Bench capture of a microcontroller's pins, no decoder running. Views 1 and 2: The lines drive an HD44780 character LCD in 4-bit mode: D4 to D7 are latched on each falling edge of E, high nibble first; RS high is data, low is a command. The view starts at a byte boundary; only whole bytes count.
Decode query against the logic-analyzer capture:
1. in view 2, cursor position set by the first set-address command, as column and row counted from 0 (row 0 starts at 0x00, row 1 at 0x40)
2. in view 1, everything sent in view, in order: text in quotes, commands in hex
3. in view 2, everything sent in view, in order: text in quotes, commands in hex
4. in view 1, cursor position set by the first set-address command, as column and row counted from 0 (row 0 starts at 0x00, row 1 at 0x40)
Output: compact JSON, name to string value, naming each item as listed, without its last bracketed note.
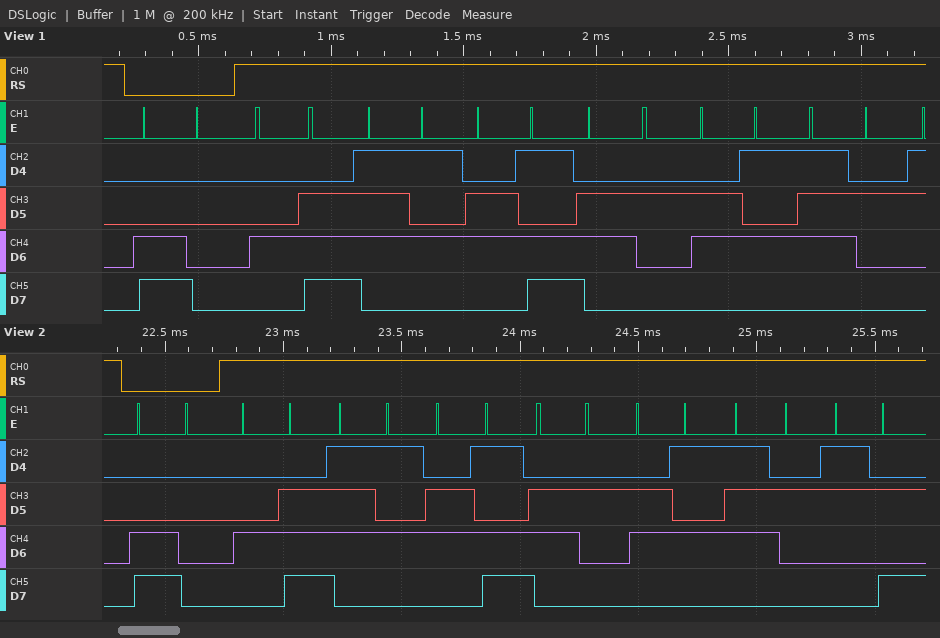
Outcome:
{"in view 2, cursor position set by the first set-address command, as column and row counted from 0": "column 0, row 1", "in view 1, everything sent in view, in order: text in quotes, commands in hex": "0xC0 \"Number\"", "in view 2, everything sent in view, in order: text in quotes, commands in hex": "0xC0 \"Number:\"", "in view 1, cursor position set by the first set-address command, as column and row counted from 0": "column 0, row 1"}
